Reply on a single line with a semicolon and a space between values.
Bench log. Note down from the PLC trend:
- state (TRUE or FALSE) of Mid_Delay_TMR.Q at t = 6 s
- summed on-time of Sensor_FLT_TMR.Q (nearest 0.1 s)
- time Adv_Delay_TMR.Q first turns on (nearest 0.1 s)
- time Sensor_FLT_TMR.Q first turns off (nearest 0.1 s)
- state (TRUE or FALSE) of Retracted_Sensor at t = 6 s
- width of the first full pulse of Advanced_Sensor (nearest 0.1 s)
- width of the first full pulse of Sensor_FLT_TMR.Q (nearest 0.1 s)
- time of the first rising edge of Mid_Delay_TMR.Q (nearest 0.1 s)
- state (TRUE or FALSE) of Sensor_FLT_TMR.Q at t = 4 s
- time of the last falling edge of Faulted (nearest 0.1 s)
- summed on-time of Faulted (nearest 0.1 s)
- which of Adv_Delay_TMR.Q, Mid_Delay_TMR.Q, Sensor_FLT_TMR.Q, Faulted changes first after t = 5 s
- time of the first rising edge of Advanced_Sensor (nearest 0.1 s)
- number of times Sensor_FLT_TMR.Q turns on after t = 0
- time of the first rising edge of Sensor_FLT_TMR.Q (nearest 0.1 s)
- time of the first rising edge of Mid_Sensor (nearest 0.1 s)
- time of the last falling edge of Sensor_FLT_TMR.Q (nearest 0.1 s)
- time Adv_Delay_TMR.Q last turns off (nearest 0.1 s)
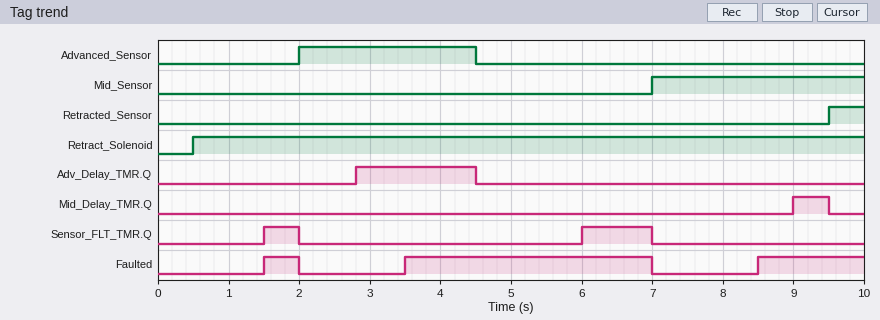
FALSE; 1.5 s; 2.8 s; 2.0 s; FALSE; 2.5 s; 0.5 s; 9.0 s; FALSE; 7.0 s; 5.5 s; Sensor_FLT_TMR.Q; 2.0 s; 2; 1.5 s; 7.0 s; 7.0 s; 4.5 s
